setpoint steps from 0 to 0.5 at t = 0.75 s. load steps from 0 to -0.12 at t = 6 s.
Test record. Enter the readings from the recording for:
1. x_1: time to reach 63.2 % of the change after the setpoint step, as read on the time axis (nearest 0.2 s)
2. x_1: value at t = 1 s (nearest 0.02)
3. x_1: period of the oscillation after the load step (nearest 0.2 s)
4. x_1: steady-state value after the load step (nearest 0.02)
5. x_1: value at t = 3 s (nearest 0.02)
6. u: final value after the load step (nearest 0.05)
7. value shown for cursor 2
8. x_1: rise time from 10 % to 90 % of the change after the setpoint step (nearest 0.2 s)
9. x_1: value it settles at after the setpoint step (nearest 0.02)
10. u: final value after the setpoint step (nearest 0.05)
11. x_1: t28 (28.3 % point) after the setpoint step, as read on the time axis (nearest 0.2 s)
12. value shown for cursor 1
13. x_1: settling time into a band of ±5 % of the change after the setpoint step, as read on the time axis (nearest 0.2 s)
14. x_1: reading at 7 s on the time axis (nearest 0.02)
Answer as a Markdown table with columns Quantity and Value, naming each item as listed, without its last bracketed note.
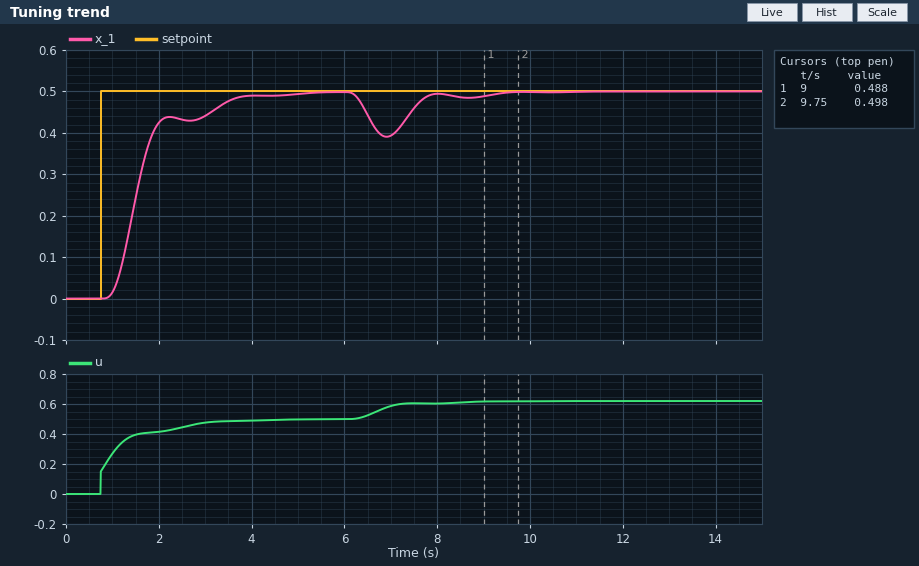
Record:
| Quantity | Value |
|---|---|
| x_1: time to reach 63.2 % of the change after the setpoint step, as read on the time axis | 1.6 s |
| x_1: value at t = 1 s | 0.02 |
| x_1: period of the oscillation after the load step | 1.8 s |
| x_1: steady-state value after the load step | 0.50 |
| x_1: value at t = 3 s | 0.44 |
| u: final value after the load step | 0.60 |
| value shown for cursor 2 | 0.498 |
| x_1: rise time from 10 % to 90 % of the change after the setpoint step | 2.0 s |
| x_1: value it settles at after the setpoint step | 0.50 |
| u: final value after the setpoint step | 0.50 |
| x_1: t28 (28.3 % point) after the setpoint step, as read on the time axis | 1.4 s |
| value shown for cursor 1 | 0.488 |
| x_1: settling time into a band of ±5 % of the change after the setpoint step, as read on the time axis | 3.4 s |
| x_1: reading at 7 s on the time axis | 0.40 |
